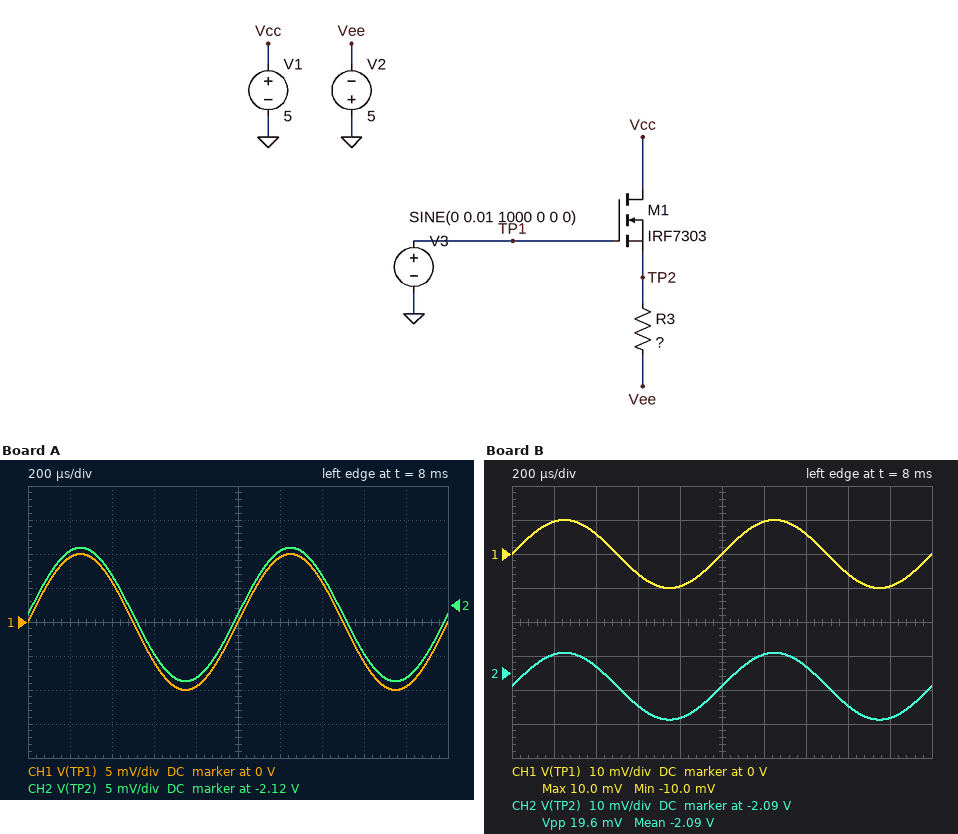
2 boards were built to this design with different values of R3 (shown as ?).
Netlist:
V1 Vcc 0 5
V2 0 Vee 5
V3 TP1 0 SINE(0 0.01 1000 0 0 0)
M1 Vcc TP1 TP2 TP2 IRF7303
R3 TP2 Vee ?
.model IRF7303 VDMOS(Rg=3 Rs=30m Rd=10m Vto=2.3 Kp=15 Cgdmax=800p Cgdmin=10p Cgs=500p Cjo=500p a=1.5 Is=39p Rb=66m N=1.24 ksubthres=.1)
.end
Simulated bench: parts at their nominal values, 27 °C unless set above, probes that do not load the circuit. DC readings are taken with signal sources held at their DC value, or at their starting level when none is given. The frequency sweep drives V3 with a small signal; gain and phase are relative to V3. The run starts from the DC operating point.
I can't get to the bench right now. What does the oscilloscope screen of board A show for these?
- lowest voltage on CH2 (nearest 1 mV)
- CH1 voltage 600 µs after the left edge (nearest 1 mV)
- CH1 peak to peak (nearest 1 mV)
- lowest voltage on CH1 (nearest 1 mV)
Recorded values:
-2.131 V
-6 mV
20 mV
-10 mV
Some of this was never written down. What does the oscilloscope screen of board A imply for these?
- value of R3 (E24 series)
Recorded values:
1.6 kΩ
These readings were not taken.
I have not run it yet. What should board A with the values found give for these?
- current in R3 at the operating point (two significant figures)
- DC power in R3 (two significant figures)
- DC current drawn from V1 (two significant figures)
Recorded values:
1.8 mA
5.2 mW
1.8 mA
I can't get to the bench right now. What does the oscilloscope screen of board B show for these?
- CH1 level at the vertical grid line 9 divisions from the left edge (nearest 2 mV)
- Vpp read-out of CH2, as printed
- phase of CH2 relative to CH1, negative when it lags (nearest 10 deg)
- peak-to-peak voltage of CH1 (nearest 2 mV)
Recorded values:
-10 mV
19.6 mV
0 deg
20 mV
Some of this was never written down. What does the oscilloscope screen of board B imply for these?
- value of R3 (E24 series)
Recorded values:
2.7 kΩ
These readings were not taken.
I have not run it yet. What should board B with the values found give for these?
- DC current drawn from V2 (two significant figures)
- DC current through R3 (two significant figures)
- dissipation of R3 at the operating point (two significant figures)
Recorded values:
1.1 mA
1.1 mA
3.1 mW
